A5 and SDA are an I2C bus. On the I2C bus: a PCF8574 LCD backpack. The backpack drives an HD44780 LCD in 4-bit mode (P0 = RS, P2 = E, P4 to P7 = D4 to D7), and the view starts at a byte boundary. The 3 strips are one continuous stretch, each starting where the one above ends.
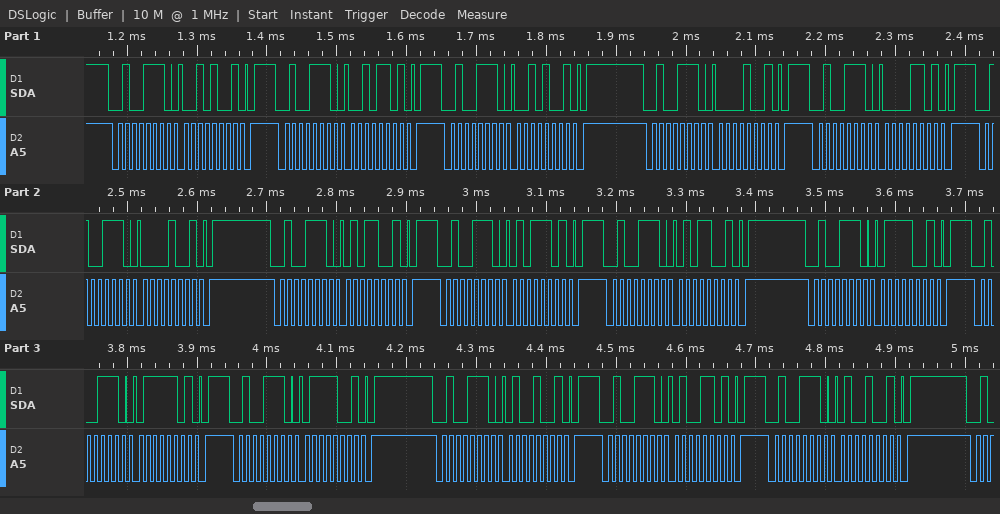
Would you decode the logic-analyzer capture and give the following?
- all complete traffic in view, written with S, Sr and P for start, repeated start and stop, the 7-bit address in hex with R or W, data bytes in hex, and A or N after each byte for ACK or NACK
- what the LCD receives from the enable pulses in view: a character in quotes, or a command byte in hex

S 27W A 29 A P S 27W A 2D A P S 27W A 29 A P S 27W A 09 A P S 27W A 0D A P S 27W A 09 A P S 27W A 59 A P S 27W A 5D A P S 27W A 59 A P S 27W A 79 A P S 27W A 7D A P S 27W A 79 A P S 27W A 49 A P S 27W A 4D A P S 27W A 49 A P
' ' 'W'
